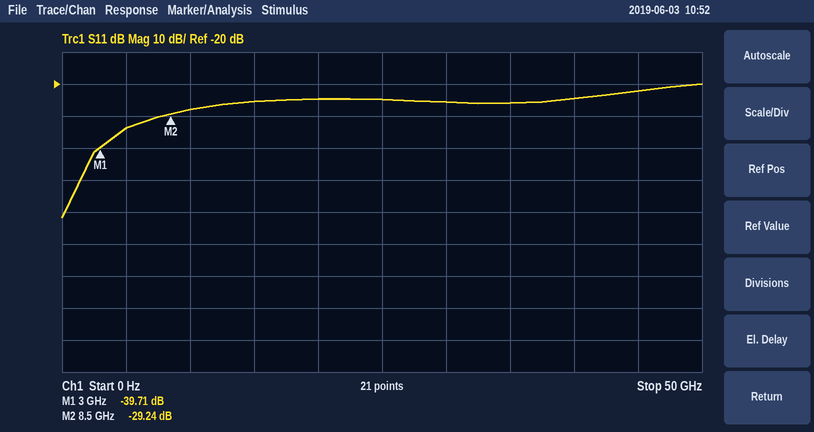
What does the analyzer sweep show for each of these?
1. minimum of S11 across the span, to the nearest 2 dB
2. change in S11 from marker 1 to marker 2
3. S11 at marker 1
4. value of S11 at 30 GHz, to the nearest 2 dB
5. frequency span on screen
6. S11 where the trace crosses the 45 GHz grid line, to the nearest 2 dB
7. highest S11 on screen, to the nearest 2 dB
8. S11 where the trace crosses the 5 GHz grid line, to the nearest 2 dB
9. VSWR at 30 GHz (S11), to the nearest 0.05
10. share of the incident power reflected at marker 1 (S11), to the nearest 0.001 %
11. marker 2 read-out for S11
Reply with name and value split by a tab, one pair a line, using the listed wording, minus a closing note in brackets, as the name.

minimum of S11 across the span, to the nearest 2 dB	-62 dB
change in S11 from marker 1 to marker 2	10.47 dB
S11 at marker 1	-39.71 dB
value of S11 at 30 GHz, to the nearest 2 dB	-26 dB
frequency span on screen	50 GHz
S11 where the trace crosses the 45 GHz grid line, to the nearest 2 dB	-22 dB
highest S11 on screen, to the nearest 2 dB	-20 dB
S11 where the trace crosses the 5 GHz grid line, to the nearest 2 dB	-34 dB
VSWR at 30 GHz (S11), to the nearest 0.05	1.10
share of the incident power reflected at marker 1 (S11), to the nearest 0.001 %	0.011 %
marker 2 read-out for S11	-29.24 dB
